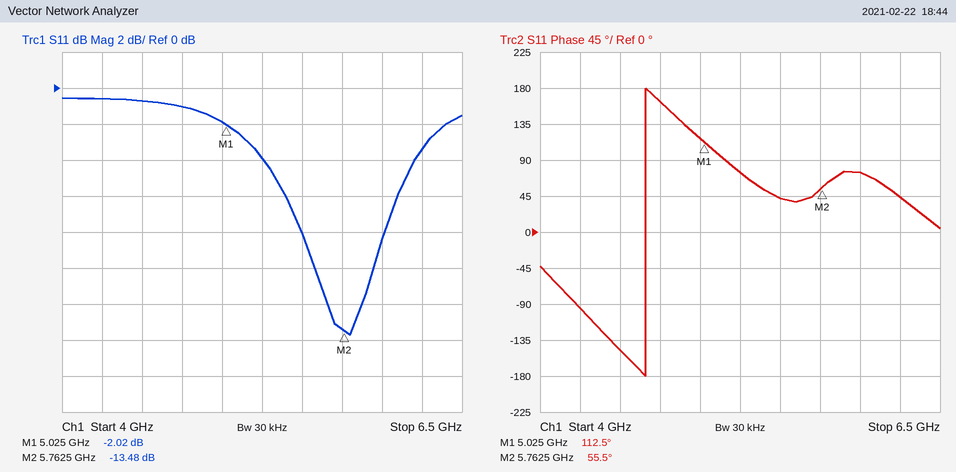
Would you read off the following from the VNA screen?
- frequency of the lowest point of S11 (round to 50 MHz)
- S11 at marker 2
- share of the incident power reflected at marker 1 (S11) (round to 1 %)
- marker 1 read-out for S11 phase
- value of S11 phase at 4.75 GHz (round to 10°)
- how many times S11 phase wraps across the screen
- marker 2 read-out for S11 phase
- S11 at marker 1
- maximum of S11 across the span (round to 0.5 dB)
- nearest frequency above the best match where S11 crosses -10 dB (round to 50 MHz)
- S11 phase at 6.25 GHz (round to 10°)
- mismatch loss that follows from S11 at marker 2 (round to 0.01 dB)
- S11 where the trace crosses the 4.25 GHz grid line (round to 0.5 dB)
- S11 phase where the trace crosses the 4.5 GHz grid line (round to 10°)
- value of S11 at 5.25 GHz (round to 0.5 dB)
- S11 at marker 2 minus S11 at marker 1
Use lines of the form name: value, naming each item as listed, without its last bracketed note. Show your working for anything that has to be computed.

frequency of the lowest point of S11: 5.80 GHz
S11 at marker 2: -13.48 dB
share of the incident power reflected at marker 1 (S11): 10^(-2.02/10) ≈ 63 %
marker 1 read-out for S11 phase: 112.5°
value of S11 phase at 4.75 GHz: 160°
how many times S11 phase wraps across the screen: 1
marker 2 read-out for S11 phase: 55.5°
S11 at marker 1: -2.02 dB
maximum of S11 across the span: -0.5 dB
nearest frequency above the best match where S11 crosses -10 dB: 5.95 GHz
S11 phase at 6.25 GHz: 40°
mismatch loss that follows from S11 at marker 2: −10 log10(1 − 10^(-13.48/10)) ≈ 0.20 dB
S11 where the trace crosses the 4.25 GHz grid line: -0.5 dB
S11 phase where the trace crosses the 4.5 GHz grid line: -150°
value of S11 at 5.25 GHz: -4.0 dB
S11 at marker 2 minus S11 at marker 1: -13.48 − (-2.02) = -11.46 dB
